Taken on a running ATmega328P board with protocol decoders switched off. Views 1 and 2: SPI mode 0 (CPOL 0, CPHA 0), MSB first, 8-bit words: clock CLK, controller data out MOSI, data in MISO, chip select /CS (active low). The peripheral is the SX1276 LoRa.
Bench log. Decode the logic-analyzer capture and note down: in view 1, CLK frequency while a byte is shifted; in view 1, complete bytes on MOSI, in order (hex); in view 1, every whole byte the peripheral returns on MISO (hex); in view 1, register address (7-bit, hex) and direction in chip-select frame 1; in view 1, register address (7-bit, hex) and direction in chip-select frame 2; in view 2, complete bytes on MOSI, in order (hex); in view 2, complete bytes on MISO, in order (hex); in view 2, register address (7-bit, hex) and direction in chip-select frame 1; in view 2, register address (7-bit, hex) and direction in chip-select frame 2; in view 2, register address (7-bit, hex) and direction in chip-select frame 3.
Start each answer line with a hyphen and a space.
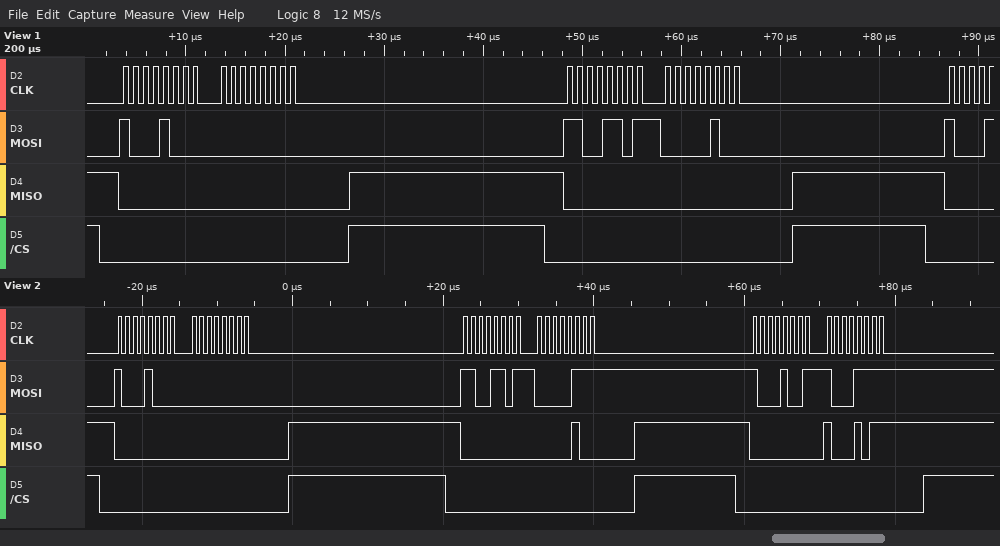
- 1 MHz
- 88 00 CD 04
- 00 00 00 00
- 0x08 write
- 0x4D write
- 0x88 0x00 0xCD 0x07 0x89 0x8F
- 0x00 0x00 0x00 0x04 0x00 0x8B
- 0x08 write
- 0x4D write
- 0x09 write
